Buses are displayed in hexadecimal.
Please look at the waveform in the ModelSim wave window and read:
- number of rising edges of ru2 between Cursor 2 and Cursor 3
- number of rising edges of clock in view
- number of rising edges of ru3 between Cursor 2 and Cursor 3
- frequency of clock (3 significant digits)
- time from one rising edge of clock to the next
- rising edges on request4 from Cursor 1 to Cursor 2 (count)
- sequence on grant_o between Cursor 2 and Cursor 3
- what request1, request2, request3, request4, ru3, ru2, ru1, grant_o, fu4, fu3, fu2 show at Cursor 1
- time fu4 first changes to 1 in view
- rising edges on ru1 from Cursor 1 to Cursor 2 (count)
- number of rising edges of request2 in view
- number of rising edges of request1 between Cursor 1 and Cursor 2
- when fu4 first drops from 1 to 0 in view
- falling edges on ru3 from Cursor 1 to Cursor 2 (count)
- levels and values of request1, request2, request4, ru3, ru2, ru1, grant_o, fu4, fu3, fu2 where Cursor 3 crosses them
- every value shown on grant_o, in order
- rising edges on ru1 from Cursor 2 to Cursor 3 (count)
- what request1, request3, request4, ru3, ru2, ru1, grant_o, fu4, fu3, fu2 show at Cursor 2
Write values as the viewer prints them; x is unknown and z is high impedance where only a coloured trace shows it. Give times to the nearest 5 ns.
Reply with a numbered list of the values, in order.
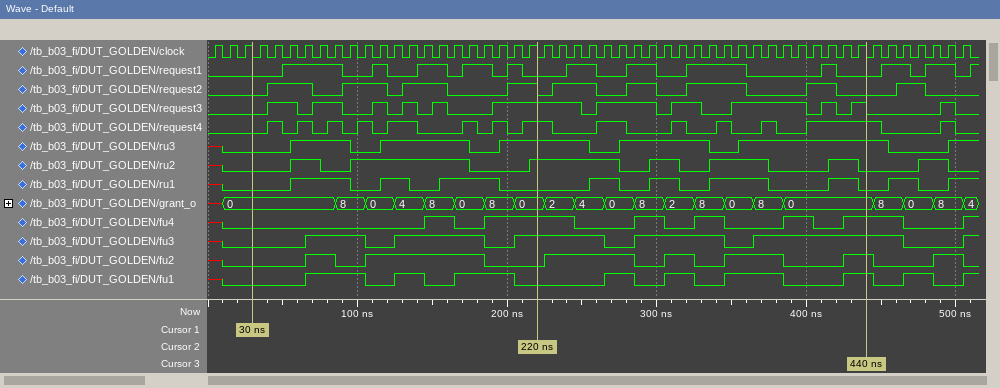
1. 3
2. 51
3. 2
4. 100 MHz
5. 10 ns
6. 8
7. 0, 2, 4, 0, 8, 2, 8, 0, 8, 0
8. request1=0, request2=0, request3=0, request4=0, ru3=0, ru2=0, ru1=0, grant_o=0, fu4=0, fu3=0, fu2=0
9. 145 ns
10. 3
11. 9
12. 5
13. 165 ns
14. 2
15. request1=0, request2=0, request4=1, ru3=1, ru2=0, ru1=0, grant_o=0, fu4=1, fu3=1, fu2=1
16. x, 0, 8, 0, 4, 8, 0, 8, 0, 2, 4, 0, 8, 2, 8, 0, 8, 0, 8, 0, 8, 4
17. 4
18. request1=0, request3=1, request4=1, ru3=1, ru2=1, ru1=0, grant_o=0, fu4=1, fu3=1, fu2=0
